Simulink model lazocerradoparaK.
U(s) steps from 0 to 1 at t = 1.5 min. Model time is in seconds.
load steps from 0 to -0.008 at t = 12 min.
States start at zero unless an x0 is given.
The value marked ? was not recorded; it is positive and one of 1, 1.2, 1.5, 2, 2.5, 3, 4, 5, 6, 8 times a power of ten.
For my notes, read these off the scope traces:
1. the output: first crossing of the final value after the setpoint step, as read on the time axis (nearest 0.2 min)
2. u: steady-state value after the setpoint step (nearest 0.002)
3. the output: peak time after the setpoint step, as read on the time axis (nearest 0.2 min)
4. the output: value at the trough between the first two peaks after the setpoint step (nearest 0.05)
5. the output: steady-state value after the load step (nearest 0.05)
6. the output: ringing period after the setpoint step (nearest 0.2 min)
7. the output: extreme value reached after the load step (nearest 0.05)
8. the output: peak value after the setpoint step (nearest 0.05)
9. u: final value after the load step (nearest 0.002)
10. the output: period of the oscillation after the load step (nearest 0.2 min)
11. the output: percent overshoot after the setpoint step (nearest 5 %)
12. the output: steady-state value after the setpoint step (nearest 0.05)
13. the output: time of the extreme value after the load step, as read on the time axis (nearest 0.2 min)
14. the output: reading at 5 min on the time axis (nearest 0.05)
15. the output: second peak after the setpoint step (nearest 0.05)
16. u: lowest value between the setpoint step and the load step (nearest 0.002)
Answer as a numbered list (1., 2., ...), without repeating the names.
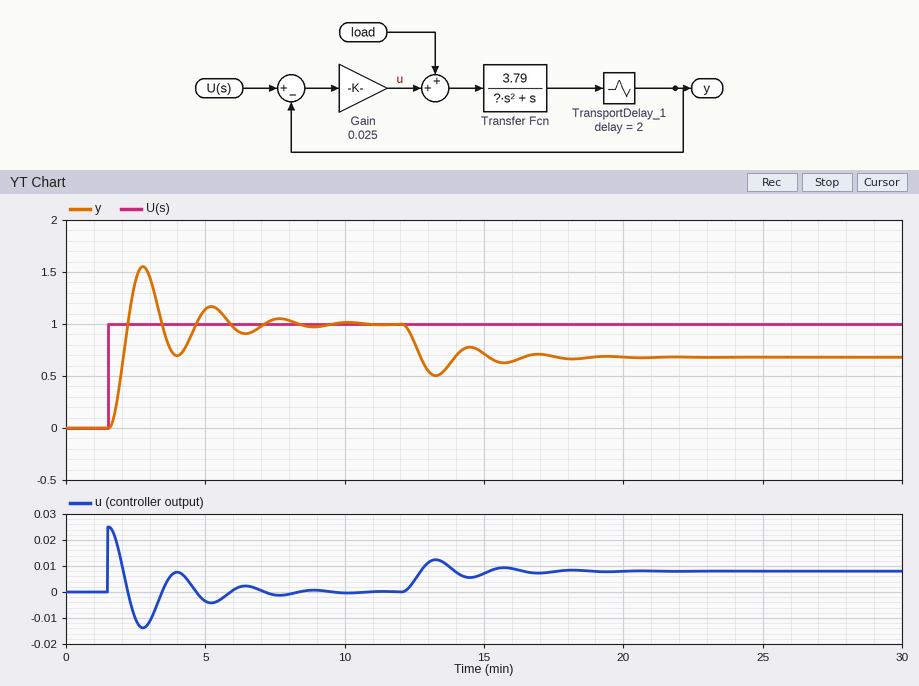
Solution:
1. 2.2 min
2. 0.000
3. 2.8 min
4. 0.70
5. 0.70
6. 2.4 min
7. 0.50
8. 1.55
9. 0.008
10. 2.4 min
11. 55 %
12. 1.00
13. 13.2 min
14. 1.15
15. 1.15
16. -0.014
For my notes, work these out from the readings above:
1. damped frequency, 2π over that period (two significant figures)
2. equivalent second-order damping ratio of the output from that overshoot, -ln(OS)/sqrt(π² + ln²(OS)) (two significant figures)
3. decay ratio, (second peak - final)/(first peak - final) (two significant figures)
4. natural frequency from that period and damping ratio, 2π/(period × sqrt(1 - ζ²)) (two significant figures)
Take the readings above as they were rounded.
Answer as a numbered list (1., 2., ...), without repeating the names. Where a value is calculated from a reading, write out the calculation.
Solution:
1. 2π / 2.4 = 2.6 rad/min
2. ln(0.55) = -0.598; 0.598 / sqrt(9.870 + 0.357) = 0.19
3. (1.15 - 1) / (1.55 - 1) = 0.27
4. 2π / (2.4 × sqrt(1 - 0.19²)) = 2.7 rad/min
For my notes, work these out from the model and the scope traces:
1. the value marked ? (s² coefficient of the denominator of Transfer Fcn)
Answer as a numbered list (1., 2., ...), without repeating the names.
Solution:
1. 50
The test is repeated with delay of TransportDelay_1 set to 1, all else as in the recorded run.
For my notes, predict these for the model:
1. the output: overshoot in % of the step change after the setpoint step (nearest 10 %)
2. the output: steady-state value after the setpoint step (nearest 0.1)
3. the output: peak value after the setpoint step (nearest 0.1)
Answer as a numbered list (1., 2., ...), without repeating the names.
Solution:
1. 50 %
2. 1.0
3. 1.5
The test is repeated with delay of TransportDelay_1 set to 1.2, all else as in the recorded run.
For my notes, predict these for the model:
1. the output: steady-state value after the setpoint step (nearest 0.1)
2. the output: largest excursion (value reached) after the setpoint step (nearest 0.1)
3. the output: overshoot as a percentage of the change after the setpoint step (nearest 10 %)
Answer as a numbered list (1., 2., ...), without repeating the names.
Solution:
1. 1.0
2. 1.5
3. 50 %
